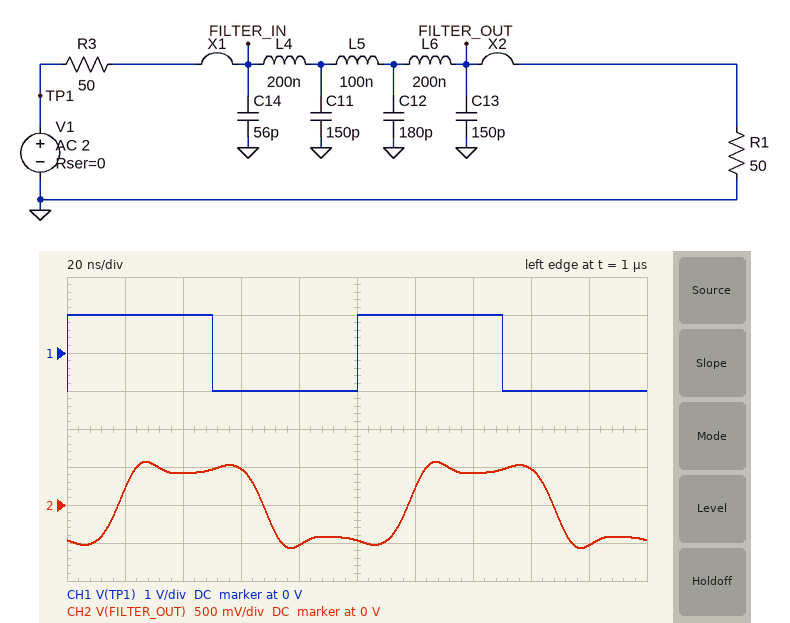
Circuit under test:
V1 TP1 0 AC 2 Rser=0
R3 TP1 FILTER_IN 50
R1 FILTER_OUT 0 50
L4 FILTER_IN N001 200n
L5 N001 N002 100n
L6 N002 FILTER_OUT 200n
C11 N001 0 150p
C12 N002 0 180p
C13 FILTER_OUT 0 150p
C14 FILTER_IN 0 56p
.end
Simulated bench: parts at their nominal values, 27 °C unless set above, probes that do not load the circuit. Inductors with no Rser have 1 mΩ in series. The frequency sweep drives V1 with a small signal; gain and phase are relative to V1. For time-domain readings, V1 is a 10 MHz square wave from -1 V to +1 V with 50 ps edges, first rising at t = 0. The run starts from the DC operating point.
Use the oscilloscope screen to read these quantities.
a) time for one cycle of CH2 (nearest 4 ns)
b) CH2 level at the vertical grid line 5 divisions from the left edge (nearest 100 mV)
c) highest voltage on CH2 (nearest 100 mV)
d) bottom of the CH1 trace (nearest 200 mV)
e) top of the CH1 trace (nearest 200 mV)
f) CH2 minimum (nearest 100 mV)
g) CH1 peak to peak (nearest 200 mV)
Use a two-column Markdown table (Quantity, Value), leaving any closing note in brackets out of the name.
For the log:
| Quantity | Value |
|---|---|
| time for one cycle of CH2 | 100 ns |
| CH2 level at the vertical grid line 5 divisions from the left edge | -500 mV |
| highest voltage on CH2 | 600 mV |
| bottom of the CH1 trace | -1.0 V |
| top of the CH1 trace | 1.0 V |
| CH2 minimum | -600 mV |
| CH1 peak to peak | 2.0 V |
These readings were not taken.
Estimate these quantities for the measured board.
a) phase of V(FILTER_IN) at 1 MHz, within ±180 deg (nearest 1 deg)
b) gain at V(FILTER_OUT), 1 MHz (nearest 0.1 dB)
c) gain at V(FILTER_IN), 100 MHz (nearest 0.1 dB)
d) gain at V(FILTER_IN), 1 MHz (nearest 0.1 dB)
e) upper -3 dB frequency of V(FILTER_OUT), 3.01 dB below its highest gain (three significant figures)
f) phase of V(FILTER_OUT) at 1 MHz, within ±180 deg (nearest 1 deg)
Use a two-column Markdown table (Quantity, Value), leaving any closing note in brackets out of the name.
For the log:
| Quantity | Value |
|---|---|
| phase of V(FILTER_IN) at 1 MHz, within ±180 deg | -3 deg |
| gain at V(FILTER_OUT), 1 MHz | -6.0 dB |
| gain at V(FILTER_IN), 100 MHz | -4.4 dB |
| gain at V(FILTER_IN), 1 MHz | -6.1 dB |
| upper -3 dB frequency of V(FILTER_OUT), 3.01 dB below its highest gain | 40.9 MHz |
| phase of V(FILTER_OUT) at 1 MHz, within ±180 deg | -7 deg |
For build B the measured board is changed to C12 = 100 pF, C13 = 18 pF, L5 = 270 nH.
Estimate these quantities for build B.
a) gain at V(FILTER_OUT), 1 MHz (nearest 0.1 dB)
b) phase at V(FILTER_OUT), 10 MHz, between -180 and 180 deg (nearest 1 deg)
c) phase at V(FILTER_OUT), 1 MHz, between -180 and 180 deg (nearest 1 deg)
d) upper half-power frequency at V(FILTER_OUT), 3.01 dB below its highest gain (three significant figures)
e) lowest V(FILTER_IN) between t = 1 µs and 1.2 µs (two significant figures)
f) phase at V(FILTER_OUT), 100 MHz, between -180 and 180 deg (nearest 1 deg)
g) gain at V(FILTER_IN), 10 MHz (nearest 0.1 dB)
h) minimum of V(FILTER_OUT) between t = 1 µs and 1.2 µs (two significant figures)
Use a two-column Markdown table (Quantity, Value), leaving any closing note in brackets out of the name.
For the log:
| Quantity | Value |
|---|---|
| gain at V(FILTER_OUT), 1 MHz | -6.0 dB |
| phase at V(FILTER_OUT), 10 MHz, between -180 and 180 deg | -54 deg |
| phase at V(FILTER_OUT), 1 MHz, between -180 and 180 deg | -5 deg |
| upper half-power frequency at V(FILTER_OUT), 3.01 dB below its highest gain | 52.6 MHz |
| lowest V(FILTER_IN) between t = 1 µs and 1.2 µs | -690 mV |
| phase at V(FILTER_OUT), 100 MHz, between -180 and 180 deg | -149 deg |
| gain at V(FILTER_IN), 10 MHz | -6.2 dB |
| minimum of V(FILTER_OUT) between t = 1 µs and 1.2 µs | -650 mV |
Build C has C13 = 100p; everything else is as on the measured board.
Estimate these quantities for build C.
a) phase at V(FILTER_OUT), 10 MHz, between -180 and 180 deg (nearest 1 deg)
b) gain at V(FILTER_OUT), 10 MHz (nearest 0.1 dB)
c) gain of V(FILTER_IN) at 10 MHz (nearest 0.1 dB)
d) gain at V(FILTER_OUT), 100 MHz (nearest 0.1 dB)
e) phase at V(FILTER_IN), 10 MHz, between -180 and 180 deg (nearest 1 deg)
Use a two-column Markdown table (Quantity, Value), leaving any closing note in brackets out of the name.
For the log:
| Quantity | Value |
|---|---|
| phase at V(FILTER_OUT), 10 MHz, between -180 and 180 deg | -59 deg |
| gain at V(FILTER_OUT), 10 MHz | -6.6 dB |
| gain of V(FILTER_IN) at 10 MHz | -9.3 dB |
| gain at V(FILTER_OUT), 100 MHz | -55.1 dB |
| phase at V(FILTER_IN), 10 MHz, between -180 and 180 deg | -13 deg |
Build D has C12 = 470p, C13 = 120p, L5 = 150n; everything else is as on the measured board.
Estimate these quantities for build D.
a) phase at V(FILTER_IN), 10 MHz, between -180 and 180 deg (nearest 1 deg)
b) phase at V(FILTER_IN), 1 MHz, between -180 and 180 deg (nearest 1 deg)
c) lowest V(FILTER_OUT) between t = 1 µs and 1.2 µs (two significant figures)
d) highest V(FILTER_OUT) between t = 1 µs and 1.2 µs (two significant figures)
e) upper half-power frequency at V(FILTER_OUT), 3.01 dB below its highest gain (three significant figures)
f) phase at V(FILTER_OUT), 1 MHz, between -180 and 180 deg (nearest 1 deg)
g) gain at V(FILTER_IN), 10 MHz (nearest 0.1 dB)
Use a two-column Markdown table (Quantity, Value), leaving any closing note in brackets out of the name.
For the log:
| Quantity | Value |
|---|---|
| phase at V(FILTER_IN), 10 MHz, between -180 and 180 deg | 1 deg |
| phase at V(FILTER_IN), 1 MHz, between -180 and 180 deg | -5 deg |
| lowest V(FILTER_OUT) between t = 1 µs and 1.2 µs | -470 mV |
| highest V(FILTER_OUT) between t = 1 µs and 1.2 µs | 470 mV |
| upper half-power frequency at V(FILTER_OUT), 3.01 dB below its highest gain | 34.1 MHz |
| phase at V(FILTER_OUT), 1 MHz, between -180 and 180 deg | -9 deg |
| gain at V(FILTER_IN), 10 MHz | -14.2 dB |
